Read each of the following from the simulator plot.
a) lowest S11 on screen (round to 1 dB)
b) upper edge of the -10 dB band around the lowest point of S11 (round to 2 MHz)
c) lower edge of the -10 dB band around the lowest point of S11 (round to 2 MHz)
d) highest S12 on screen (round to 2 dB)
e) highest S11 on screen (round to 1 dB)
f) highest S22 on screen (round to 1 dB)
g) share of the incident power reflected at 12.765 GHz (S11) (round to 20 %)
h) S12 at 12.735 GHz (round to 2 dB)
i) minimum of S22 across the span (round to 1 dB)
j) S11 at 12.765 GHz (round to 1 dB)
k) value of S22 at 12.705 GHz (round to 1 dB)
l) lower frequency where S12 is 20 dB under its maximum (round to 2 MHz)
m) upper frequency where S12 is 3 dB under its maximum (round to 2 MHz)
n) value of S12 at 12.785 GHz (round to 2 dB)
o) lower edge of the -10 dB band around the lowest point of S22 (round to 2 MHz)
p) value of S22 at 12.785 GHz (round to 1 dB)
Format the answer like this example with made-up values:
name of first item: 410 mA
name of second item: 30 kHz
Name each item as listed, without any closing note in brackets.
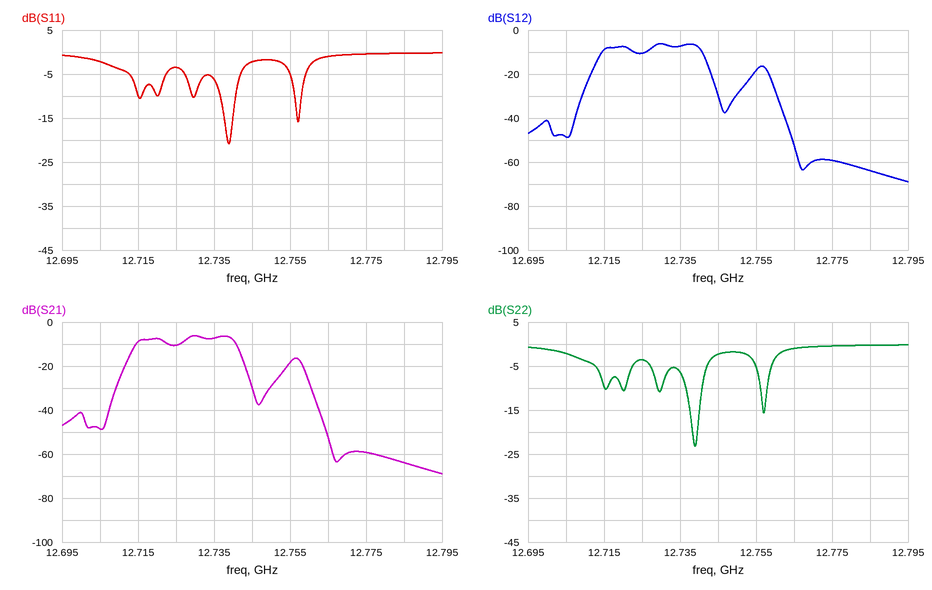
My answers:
lowest S11 on screen: -21 dB
upper edge of the -10 dB band around the lowest point of S11: 12.740 GHz
lower edge of the -10 dB band around the lowest point of S11: 12.736 GHz
highest S12 on screen: -6 dB
highest S11 on screen: 0 dB
highest S22 on screen: 0 dB
share of the incident power reflected at 12.765 GHz (S11): 80 %
S12 at 12.735 GHz: -8 dB
minimum of S22 across the span: -23 dB
S11 at 12.765 GHz: -1 dB
value of S22 at 12.705 GHz: -2 dB
lower frequency where S12 is 20 dB under its maximum: 12.710 GHz
upper frequency where S12 is 3 dB under its maximum: 12.740 GHz
value of S12 at 12.785 GHz: -64 dB
lower edge of the -10 dB band around the lowest point of S22: 12.736 GHz
value of S22 at 12.785 GHz: 0 dB
